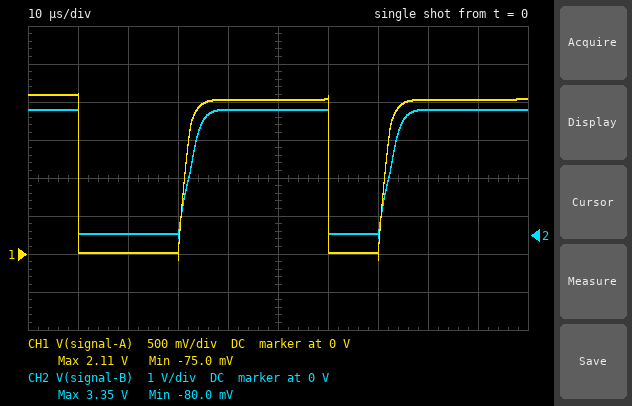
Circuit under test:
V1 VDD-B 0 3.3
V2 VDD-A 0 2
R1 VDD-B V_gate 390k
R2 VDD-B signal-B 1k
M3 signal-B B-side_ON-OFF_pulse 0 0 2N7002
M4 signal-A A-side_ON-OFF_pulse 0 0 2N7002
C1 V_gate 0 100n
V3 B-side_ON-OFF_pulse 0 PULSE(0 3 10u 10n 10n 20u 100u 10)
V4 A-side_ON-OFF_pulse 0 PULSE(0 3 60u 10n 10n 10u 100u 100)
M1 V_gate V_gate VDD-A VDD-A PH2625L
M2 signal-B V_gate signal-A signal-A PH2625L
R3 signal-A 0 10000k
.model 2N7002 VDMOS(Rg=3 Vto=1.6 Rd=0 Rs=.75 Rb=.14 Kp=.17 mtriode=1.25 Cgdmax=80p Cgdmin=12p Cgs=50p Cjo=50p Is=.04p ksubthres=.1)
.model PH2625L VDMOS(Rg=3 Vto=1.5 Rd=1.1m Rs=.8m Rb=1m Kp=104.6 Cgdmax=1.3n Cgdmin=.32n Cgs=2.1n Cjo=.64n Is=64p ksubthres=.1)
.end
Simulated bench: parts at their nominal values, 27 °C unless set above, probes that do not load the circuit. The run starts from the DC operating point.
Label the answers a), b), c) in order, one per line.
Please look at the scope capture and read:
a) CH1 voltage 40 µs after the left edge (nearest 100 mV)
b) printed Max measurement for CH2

a) 2.0 V
b) 3.35 V
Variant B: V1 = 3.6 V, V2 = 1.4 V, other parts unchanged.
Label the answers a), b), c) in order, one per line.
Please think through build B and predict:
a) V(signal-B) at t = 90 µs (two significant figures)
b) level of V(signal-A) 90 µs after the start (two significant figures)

a) 3.6 V
b) 1.6 V
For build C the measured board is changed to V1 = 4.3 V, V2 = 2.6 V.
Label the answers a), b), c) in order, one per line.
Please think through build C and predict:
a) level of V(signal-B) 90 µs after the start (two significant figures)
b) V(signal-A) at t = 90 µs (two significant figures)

a) 4.3 V
b) 2.7 V
